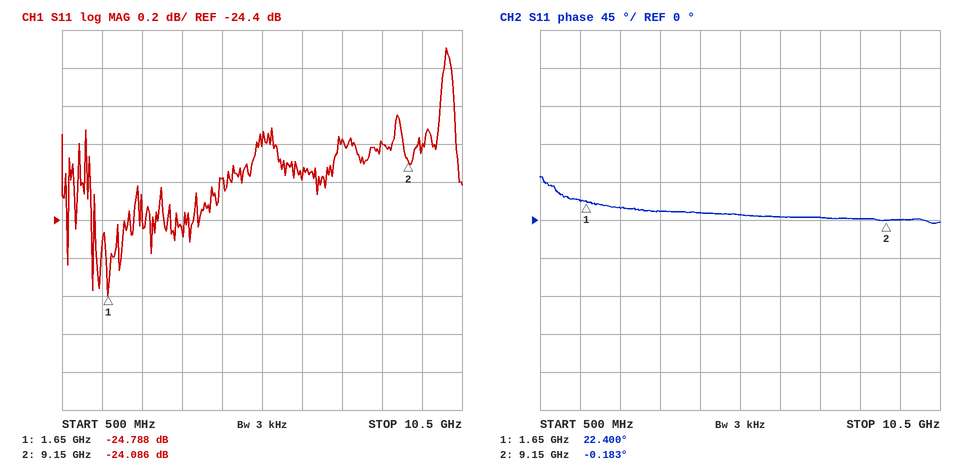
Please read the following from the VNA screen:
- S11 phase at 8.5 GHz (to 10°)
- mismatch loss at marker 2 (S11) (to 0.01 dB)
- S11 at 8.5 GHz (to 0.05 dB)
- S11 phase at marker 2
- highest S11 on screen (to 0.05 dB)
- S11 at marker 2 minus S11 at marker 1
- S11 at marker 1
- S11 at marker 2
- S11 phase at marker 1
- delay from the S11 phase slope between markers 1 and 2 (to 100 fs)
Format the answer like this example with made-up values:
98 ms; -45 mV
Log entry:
0°; 0.02 dB; -24.00 dB; -0.183°; -23.50 dB; 0.702 dB; -24.788 dB; -24.086 dB; 22.400°; 8.4 ps
